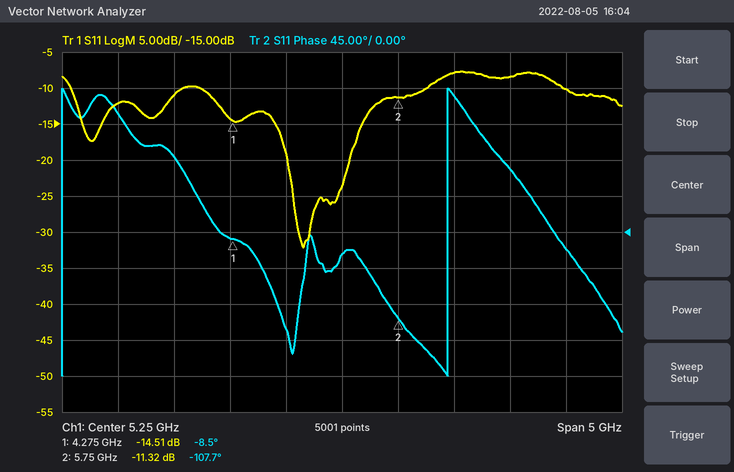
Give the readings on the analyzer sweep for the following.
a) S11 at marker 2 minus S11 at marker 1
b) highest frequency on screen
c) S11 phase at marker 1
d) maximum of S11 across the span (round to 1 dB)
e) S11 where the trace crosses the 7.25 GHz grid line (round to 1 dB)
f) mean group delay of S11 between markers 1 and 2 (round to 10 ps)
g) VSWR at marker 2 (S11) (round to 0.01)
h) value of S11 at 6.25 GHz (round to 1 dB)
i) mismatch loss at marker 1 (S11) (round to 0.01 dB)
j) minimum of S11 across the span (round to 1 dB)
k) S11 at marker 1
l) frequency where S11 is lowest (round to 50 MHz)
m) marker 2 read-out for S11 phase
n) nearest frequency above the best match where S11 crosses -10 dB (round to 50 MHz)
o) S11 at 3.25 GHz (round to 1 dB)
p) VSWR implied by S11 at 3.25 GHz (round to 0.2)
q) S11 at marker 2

3.19 dB
7.75 GHz
-8.5°
-8 dB
-10 dB
190 ps
1.75
-8 dB
0.16 dB
-32 dB
-14.51 dB
4.90 GHz
-107.7°
6.00 GHz
-12 dB
1.6
-11.32 dB
